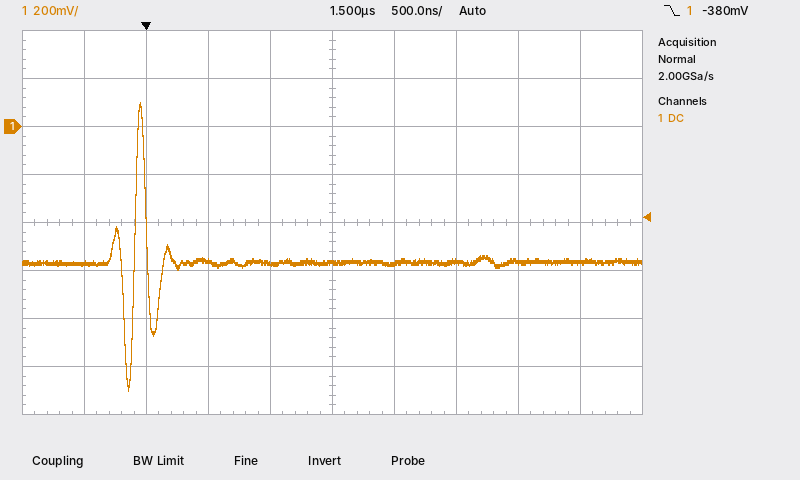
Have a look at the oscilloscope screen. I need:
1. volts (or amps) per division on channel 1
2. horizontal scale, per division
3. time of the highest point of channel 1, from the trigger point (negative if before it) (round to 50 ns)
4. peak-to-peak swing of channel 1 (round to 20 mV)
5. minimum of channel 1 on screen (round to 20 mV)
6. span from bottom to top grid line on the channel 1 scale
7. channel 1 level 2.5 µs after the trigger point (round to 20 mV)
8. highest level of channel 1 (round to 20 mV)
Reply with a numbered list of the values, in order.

1. 200 mV
2. 500 ns
3. -50 ns
4. 1.20 V
5. -1.10 V
6. 1.6 V
7. -560 mV
8. 100 mV
